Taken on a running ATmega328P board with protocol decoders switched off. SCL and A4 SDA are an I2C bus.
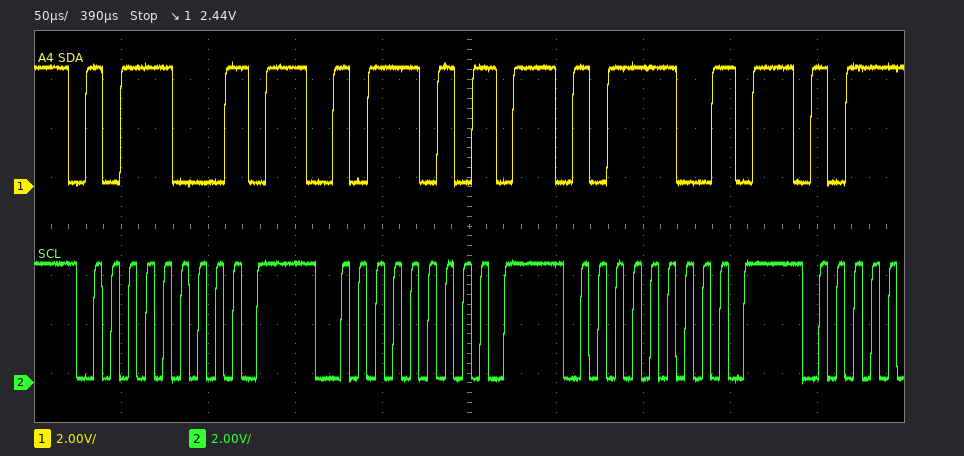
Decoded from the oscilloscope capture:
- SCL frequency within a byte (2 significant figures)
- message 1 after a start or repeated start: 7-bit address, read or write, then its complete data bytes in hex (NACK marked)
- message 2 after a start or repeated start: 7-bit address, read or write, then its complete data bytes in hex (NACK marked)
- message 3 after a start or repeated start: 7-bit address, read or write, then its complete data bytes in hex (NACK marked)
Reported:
100 kHz
0x5C write NACK
0x5D write NACK
0x5E write NACK
